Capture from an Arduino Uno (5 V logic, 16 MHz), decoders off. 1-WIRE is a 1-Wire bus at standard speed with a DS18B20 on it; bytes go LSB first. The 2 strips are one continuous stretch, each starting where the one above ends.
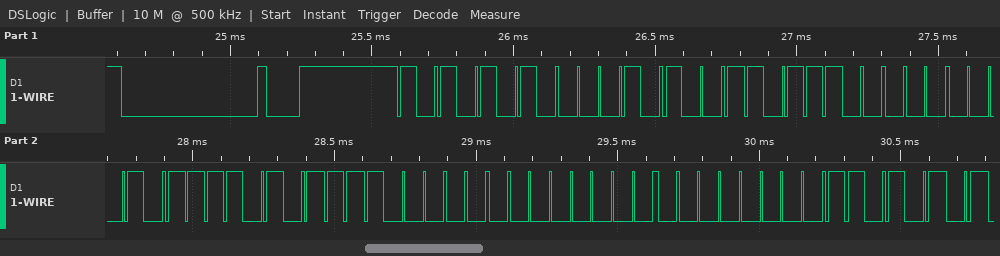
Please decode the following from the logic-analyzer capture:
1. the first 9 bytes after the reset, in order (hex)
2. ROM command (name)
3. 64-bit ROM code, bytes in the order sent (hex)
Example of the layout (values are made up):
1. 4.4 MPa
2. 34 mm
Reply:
1. 55 28 3B 40 AF 07 00 00 AB
2. Match ROM
3. 28 3B 40 AF 07 00 00 AB
